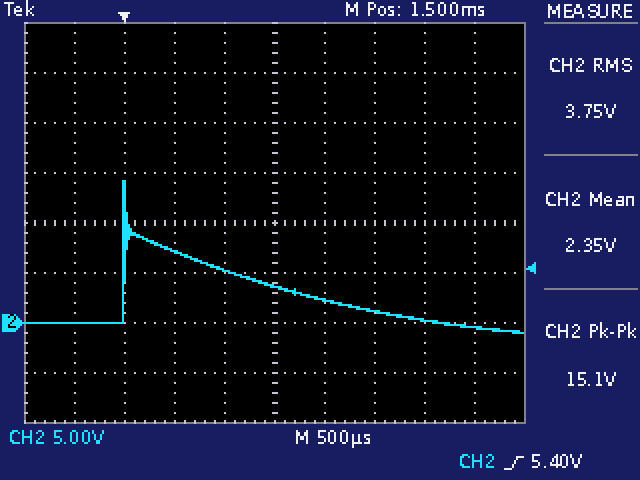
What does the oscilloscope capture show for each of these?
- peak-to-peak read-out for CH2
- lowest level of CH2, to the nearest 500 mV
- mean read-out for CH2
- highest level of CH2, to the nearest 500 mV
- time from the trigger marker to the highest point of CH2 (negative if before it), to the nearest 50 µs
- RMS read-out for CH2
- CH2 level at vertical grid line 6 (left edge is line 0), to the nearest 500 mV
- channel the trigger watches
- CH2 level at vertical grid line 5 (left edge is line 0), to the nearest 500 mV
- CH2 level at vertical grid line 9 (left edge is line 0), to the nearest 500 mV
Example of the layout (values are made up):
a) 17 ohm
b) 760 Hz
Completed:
a) 15.1 V
b) -1.0 V
c) 2.35 V
d) 14.0 V
e) 0 µs
f) 3.75 V
g) 2.5 V
h) CH2
i) 3.5 V
j) -500 mV
